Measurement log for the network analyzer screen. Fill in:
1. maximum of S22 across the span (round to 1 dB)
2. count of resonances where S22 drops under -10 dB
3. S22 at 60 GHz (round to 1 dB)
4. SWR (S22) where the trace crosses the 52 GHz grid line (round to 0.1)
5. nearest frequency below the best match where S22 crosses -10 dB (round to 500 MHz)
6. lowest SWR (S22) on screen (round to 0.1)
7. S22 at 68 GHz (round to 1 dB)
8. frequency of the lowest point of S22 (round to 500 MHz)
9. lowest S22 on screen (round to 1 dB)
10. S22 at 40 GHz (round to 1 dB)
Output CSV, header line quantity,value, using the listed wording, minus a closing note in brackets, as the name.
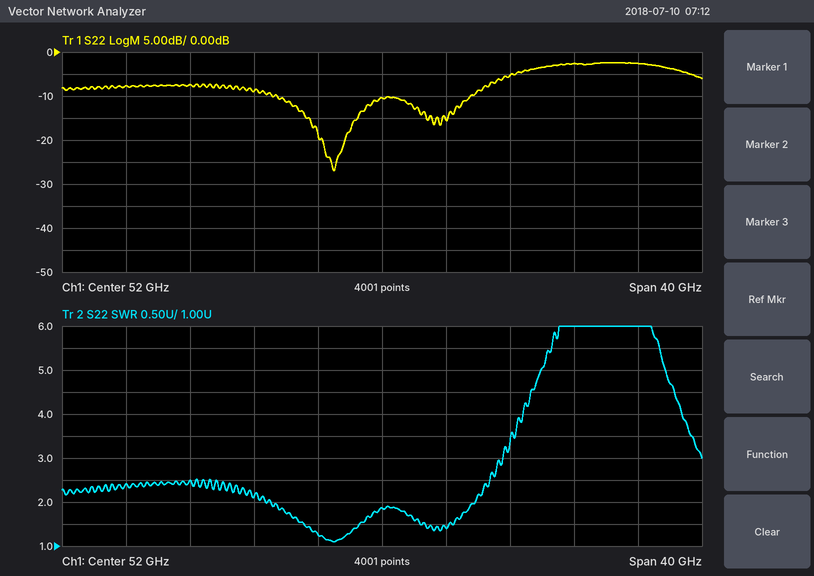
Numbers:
quantity,value
maximum of S22 across the span,-2 dB
count of resonances where S22 drops under -10 dB,2
S22 at 60 GHz,-5 dB
SWR (S22) where the trace crosses the 52 GHz grid line,1.9
nearest frequency below the best match where S22 crosses -10 dB,45.5 GHz
lowest SWR (S22) on screen,1.1
S22 at 68 GHz,-3 dB
frequency of the lowest point of S22,49.0 GHz
lowest S22 on screen,-27 dB
S22 at 40 GHz,-7 dB
